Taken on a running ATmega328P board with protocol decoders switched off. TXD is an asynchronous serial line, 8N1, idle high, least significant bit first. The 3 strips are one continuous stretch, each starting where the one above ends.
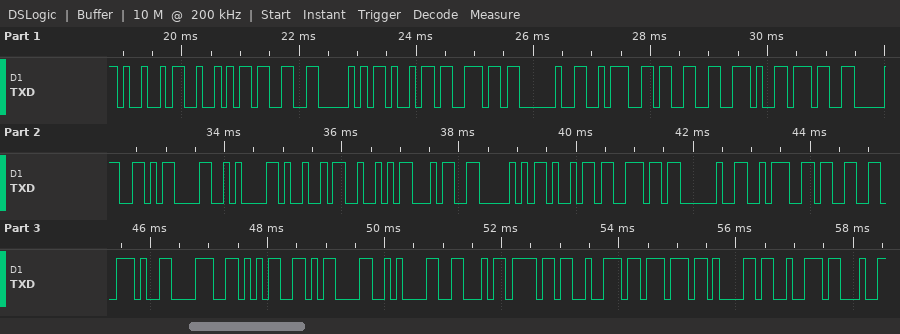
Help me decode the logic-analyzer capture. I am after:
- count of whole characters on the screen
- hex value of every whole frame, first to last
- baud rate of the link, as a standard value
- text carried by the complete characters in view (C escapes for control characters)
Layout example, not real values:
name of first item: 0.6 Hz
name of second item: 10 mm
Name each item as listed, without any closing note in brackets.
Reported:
count of whole characters on the screen: 34
hex value of every whole frame, first to last: 49 52 33 50 69 6E 20 3A 33 2E 37 30 0D 0A 49 52 34 50 69 6E 20 3A 33 2E 38 35 0D 0A 46 6F 72 77 61 72
baud rate of the link, as a standard value: 9600 baud
text carried by the complete characters in view: "IR3Pin :3.70\r\nIR4Pin :3.85\r\nForwar"
